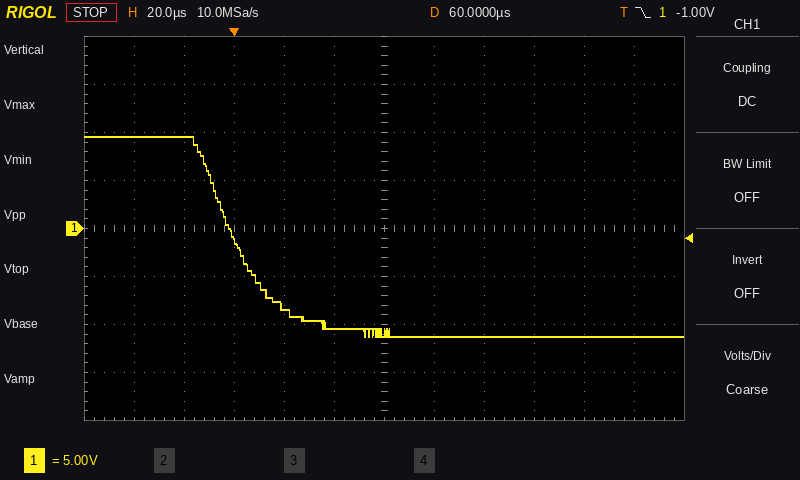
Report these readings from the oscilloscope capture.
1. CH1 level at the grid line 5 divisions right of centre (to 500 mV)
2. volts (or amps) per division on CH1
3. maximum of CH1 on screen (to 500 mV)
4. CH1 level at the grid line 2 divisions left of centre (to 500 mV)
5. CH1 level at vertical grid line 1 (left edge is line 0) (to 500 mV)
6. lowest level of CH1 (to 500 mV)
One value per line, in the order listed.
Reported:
-11.0 V
5 V
9.5 V
-8.0 V
9.5 V
-11.0 V
